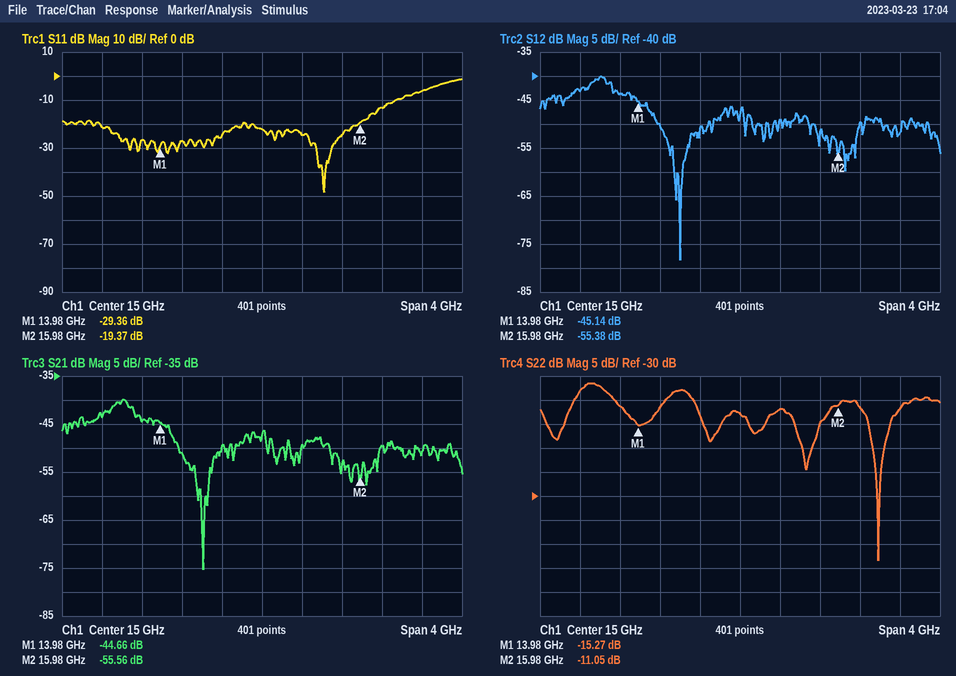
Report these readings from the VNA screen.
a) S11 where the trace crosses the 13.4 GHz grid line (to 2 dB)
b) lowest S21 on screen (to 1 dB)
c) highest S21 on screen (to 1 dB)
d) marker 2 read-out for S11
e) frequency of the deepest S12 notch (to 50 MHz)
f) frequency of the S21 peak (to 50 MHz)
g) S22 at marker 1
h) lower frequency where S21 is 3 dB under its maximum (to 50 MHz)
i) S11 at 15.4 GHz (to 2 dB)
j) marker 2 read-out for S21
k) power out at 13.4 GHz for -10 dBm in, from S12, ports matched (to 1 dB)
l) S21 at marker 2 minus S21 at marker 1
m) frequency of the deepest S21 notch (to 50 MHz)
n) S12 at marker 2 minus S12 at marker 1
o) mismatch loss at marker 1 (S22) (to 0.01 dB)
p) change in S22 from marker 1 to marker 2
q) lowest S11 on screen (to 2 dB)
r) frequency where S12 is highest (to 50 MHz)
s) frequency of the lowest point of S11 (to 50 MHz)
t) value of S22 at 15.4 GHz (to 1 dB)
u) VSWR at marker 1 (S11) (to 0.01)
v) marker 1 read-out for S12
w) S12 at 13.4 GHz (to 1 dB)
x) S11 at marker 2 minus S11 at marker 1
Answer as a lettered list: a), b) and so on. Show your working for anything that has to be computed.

a) -22 dB
b) -75 dB
c) -40 dB
d) -19.37 dB
e) 14.40 GHz
f) 13.60 GHz
g) -15.27 dB
h) 13.40 GHz
i) -24 dB
j) -55.56 dB
k) -10 dBm + (-43 dB) = -53 dBm
l) -55.56 − (-44.66) = -10.90 dB
m) 14.40 GHz
n) -55.38 − (-45.14) = -10.24 dB
o) −10 log10(1 − 10^(-15.27/10)) ≈ 0.13 dB
p) -11.05 − (-15.27) = 4.22 dB
q) -48 dB
r) 13.60 GHz
s) 15.60 GHz
t) -12 dB
u) (1 + 0.0340)/(1 − 0.0340) ≈ 1.07
v) -45.14 dB
w) -43 dB
x) -19.37 − (-29.36) = 9.99 dB
